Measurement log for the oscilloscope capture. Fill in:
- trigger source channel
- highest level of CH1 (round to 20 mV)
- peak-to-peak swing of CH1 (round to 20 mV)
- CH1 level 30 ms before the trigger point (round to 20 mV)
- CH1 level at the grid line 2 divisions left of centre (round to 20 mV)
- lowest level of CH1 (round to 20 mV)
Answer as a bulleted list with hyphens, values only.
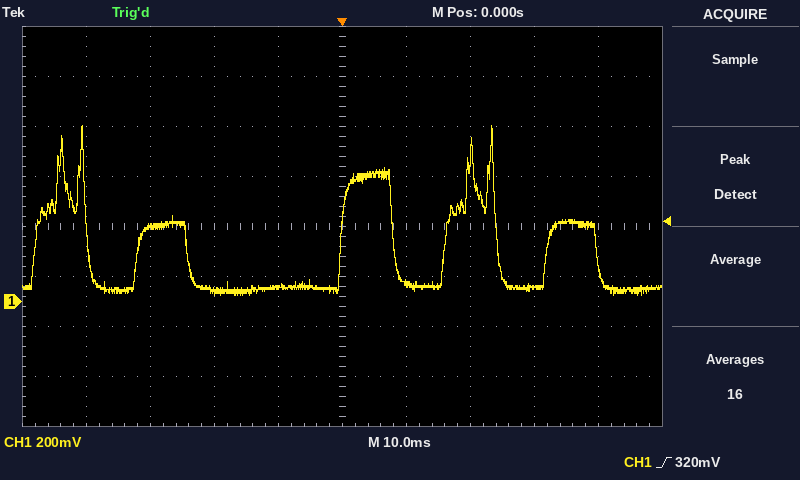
- CH1
- 700 mV
- 680 mV
- 300 mV
- 40 mV
- 20 mV
